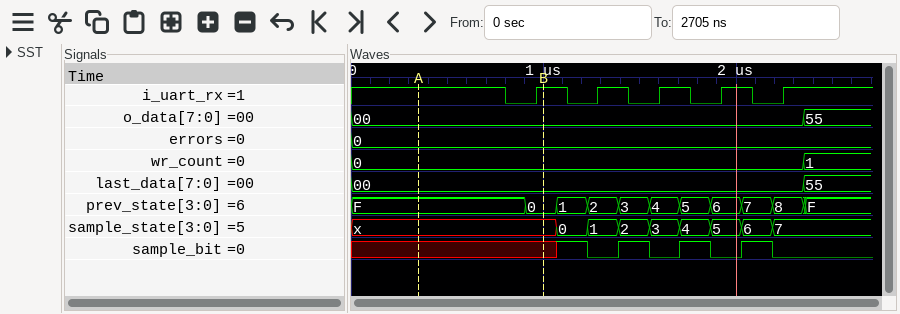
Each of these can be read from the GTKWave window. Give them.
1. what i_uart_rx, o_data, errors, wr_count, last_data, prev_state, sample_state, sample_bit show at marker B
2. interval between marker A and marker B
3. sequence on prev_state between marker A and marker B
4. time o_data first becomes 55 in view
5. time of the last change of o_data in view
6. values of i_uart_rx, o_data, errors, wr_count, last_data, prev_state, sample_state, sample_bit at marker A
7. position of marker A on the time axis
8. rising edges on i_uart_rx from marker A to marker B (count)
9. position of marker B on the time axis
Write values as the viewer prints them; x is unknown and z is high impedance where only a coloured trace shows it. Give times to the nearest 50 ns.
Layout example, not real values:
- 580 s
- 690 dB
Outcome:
- i_uart_rx=1, o_data=00, errors=0, wr_count=0, last_data=00, prev_state=0, sample_state=x, sample_bit=x
- 650 ns
- F, 0
- 2350 ns
- 2350 ns
- i_uart_rx=1, o_data=00, errors=0, wr_count=0, last_data=00, prev_state=F, sample_state=x, sample_bit=x
- 350 ns
- 1
- 1000 ns
